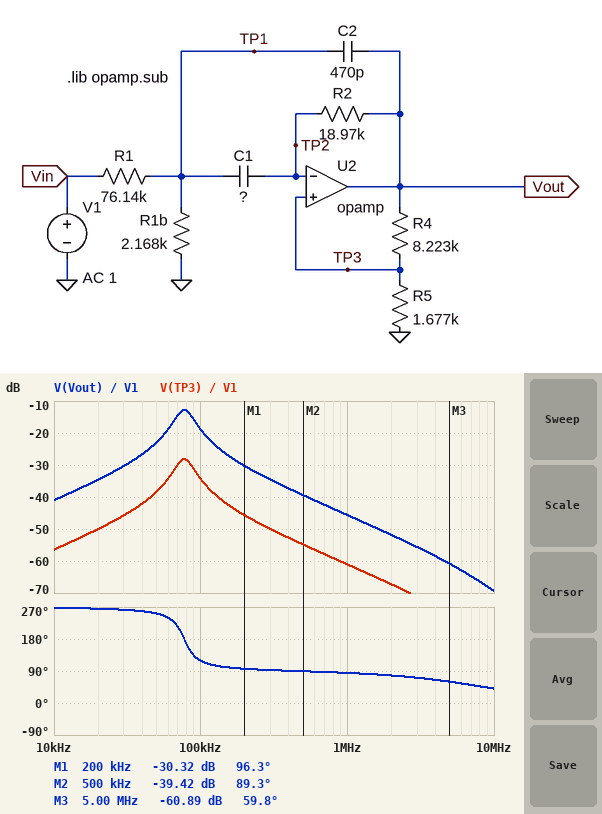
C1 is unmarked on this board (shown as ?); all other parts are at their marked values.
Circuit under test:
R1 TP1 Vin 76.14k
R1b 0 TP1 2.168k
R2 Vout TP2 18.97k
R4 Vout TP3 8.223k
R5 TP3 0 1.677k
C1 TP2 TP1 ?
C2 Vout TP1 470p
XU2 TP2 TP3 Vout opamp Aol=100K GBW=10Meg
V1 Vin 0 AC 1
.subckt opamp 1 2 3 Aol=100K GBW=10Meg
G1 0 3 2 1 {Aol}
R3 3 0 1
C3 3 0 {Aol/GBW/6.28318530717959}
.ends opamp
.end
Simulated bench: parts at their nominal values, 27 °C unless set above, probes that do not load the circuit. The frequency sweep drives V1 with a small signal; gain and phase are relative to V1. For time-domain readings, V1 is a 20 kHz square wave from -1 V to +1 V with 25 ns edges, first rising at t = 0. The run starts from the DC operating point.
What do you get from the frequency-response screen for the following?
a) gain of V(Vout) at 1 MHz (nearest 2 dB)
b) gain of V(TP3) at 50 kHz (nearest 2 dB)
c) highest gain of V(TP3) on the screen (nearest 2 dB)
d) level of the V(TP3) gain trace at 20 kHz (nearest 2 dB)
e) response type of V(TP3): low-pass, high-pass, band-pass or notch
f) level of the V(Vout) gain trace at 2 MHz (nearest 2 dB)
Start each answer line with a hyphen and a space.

- -46 dB
- -38 dB
- -28 dB
- -50 dB
- band-pass
- -52 dB
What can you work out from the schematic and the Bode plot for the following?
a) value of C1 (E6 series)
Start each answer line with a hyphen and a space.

- 220 pF
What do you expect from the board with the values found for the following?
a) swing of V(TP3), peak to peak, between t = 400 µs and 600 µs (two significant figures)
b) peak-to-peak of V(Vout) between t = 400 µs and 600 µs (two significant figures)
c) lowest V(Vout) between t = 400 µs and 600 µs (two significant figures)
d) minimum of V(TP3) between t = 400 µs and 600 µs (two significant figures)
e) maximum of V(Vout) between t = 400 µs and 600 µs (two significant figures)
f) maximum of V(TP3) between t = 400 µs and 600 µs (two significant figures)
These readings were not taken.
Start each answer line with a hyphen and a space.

- 33 mV
- 190 mV
- -97 mV
- -16 mV
- 97 mV
- 16 mV
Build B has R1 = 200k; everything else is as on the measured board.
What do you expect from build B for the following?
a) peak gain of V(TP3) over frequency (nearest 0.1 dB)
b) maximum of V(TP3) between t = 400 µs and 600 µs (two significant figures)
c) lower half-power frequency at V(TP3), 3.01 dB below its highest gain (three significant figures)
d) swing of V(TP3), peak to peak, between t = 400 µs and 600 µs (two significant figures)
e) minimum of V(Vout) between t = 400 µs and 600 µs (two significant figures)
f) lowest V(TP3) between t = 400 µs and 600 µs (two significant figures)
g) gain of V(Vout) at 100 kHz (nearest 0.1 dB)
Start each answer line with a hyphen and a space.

- -36.8 dB
- 6.3 mV
- 66.0 kHz
- 13 mV
- -37 mV
- -6.3 mV
- -27.5 dB
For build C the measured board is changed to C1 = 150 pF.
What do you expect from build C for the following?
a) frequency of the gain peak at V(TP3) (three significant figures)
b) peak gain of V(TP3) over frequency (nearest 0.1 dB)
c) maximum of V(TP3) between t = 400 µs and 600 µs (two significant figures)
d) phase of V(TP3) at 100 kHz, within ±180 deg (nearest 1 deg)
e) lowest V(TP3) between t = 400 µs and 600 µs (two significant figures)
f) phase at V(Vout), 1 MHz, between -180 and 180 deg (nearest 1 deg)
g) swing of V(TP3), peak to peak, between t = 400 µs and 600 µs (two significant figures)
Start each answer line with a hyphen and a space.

- 93.7 kHz
- -33.1 dB
- 14 mV
- 162 deg
- -14 mV
- 86 deg
- 28 mV
